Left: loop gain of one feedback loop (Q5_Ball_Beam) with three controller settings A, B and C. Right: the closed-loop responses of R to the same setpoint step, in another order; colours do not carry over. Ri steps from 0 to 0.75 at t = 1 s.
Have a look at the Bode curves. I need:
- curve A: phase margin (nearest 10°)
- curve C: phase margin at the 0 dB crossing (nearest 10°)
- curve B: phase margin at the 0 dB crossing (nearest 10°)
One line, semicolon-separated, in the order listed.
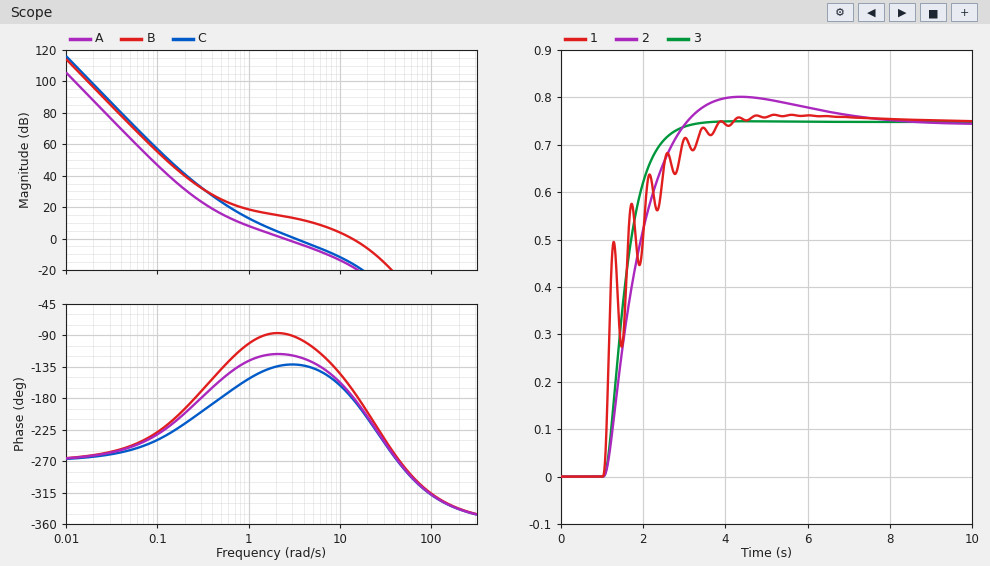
60°; 50°; 10°
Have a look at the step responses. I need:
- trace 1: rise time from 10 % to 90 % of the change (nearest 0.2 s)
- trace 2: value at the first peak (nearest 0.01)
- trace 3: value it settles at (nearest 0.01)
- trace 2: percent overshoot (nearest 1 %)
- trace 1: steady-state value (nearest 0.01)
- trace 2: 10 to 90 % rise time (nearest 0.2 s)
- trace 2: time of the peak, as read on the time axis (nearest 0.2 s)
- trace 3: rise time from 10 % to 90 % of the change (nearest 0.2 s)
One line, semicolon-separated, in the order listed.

1.4 s; 0.80; 0.75; 7 %; 0.75; 1.4 s; 4.4 s; 1.0 s
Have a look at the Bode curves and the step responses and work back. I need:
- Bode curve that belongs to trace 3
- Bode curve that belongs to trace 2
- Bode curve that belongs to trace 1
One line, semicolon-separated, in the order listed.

C; A; B
